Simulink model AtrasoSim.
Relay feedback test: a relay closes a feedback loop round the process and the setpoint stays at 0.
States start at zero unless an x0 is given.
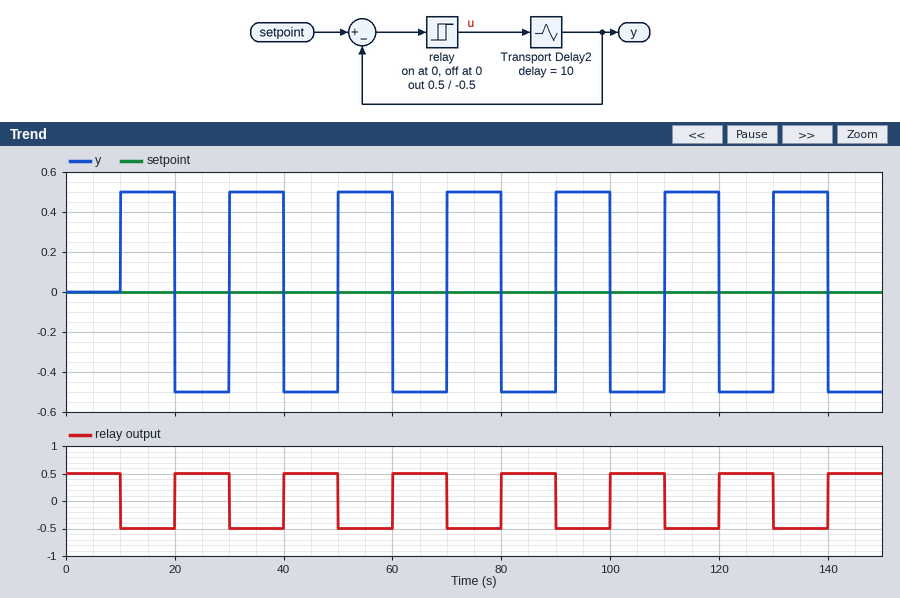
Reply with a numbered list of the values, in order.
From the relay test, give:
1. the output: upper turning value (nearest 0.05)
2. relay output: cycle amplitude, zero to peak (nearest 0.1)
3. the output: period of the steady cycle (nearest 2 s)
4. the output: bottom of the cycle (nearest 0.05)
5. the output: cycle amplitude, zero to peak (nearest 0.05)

1. 0.50
2. 0.5
3. 20 s
4. -0.50
5. 0.50
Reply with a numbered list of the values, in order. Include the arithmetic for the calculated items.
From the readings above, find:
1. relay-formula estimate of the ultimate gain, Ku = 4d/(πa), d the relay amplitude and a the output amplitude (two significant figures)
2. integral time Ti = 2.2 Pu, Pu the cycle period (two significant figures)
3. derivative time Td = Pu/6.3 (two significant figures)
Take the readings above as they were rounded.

1. 4 × 0.5 / (π × 0.5) = 1.3
2. 2.2 × 20 = 44 s
3. 20 / 6.3 = 3.2 s
